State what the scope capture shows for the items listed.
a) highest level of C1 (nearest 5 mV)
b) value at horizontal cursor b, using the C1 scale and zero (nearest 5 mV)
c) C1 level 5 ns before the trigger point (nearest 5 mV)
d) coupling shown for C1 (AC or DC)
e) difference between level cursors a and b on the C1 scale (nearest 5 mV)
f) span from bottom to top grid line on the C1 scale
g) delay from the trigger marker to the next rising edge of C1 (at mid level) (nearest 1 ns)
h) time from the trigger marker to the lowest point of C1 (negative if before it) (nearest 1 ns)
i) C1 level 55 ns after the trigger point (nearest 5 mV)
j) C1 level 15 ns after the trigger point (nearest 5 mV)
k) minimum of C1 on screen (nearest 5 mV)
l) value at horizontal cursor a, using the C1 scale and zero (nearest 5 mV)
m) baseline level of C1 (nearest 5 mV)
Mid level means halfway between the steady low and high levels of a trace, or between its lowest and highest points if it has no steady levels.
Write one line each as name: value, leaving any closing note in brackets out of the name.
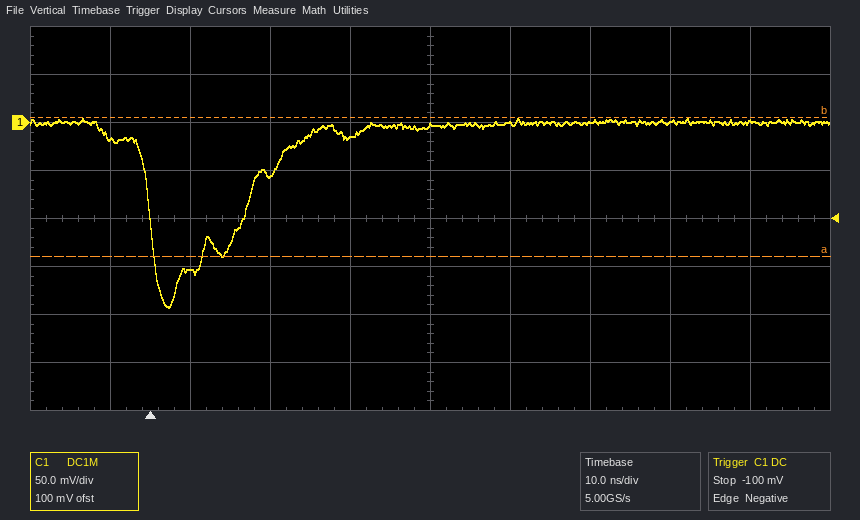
highest level of C1: 5 mV
value at horizontal cursor b, using the C1 scale and zero: 5 mV
C1 level 5 ns before the trigger point: -15 mV
coupling shown for C1: DC
difference between level cursors a and b on the C1 scale: 145 mV
span from bottom to top grid line on the C1 scale: 400 mV
delay from the trigger marker to the next rising edge of C1 (at mid level): 12 ns
time from the trigger marker to the lowest point of C1 (negative if before it): +2 ns
C1 level 55 ns after the trigger point: 0 mV
C1 level 15 ns after the trigger point: -55 mV
minimum of C1 on screen: -195 mV
value at horizontal cursor a, using the C1 scale and zero: -140 mV
baseline level of C1: 0 mV
